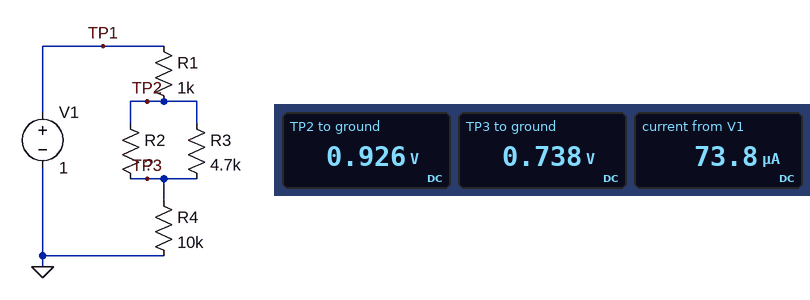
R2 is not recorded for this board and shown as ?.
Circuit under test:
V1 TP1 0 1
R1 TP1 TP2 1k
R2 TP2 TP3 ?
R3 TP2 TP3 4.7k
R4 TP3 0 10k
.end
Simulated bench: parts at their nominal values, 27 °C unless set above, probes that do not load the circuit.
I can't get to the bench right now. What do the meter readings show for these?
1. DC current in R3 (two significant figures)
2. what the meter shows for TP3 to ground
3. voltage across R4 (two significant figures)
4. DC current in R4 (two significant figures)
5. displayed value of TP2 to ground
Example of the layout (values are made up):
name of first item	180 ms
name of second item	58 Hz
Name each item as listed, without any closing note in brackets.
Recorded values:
DC current in R3	40 µA
what the meter shows for TP3 to ground	0.738 V
voltage across R4	740 mV
DC current in R4	74 µA
displayed value of TP2 to ground	0.926 V
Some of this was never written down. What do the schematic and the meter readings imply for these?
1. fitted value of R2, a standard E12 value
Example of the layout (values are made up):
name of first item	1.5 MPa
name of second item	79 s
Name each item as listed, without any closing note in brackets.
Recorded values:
fitted value of R2, a standard E12 value	5.6 kΩ
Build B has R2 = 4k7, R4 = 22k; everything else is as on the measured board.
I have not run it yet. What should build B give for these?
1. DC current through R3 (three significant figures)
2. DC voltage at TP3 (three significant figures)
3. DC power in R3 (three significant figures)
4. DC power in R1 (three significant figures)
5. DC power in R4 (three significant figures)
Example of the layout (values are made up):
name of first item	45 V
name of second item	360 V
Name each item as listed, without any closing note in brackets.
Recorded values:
DC current through R3	19.7 µA
DC voltage at TP3	868 mV
DC power in R3	1.83 µW
DC power in R1	1.56 µW
DC power in R4	34.2 µW
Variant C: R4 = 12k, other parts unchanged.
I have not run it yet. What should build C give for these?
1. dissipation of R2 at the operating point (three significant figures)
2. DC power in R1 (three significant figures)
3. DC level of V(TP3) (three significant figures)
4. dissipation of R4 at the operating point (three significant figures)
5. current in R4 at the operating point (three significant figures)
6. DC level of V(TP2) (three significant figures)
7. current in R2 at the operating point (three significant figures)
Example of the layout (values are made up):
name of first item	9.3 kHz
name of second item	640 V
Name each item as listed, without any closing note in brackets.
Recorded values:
dissipation of R2 at the operating point	4.82 µW
DC power in R1	4.13 µW
DC level of V(TP3)	771 mV
dissipation of R4 at the operating point	49.6 µW
current in R4 at the operating point	64.3 µA
DC level of V(TP2)	936 mV
current in R2 at the operating point	29.3 µA
